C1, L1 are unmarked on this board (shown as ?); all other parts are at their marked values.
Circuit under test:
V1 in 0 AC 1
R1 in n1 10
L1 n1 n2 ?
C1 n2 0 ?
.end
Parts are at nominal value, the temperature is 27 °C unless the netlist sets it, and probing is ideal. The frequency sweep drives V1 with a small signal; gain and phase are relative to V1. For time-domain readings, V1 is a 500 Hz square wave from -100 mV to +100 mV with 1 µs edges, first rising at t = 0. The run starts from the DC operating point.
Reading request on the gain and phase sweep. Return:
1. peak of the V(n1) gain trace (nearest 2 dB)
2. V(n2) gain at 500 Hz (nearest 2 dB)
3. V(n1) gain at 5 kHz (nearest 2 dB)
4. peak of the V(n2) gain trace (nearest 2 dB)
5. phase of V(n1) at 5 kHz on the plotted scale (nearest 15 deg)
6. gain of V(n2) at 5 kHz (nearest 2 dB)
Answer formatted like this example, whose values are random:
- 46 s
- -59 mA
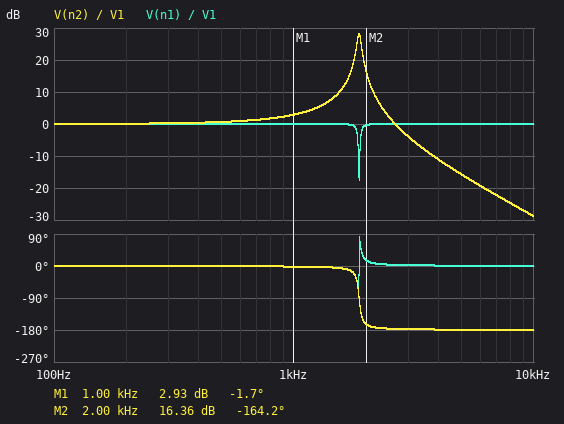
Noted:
- 0 dB
- 0 dB
- 0 dB
- 28 dB
- 0 deg
- -16 dB
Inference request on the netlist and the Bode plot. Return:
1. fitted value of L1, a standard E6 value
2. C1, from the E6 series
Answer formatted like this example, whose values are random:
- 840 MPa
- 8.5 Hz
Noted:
- 22 mH
- 330 nF
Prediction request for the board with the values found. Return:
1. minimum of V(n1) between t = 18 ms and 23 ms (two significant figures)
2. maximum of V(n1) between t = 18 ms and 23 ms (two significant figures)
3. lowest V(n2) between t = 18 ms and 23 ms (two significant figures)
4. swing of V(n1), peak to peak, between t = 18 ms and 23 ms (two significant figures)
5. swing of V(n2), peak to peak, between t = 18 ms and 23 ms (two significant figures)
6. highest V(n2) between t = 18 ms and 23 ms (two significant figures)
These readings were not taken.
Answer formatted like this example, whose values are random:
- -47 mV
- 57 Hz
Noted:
- -100 mV
- 100 mV
- -220 mV
- 210 mV
- 430 mV
- 220 mV
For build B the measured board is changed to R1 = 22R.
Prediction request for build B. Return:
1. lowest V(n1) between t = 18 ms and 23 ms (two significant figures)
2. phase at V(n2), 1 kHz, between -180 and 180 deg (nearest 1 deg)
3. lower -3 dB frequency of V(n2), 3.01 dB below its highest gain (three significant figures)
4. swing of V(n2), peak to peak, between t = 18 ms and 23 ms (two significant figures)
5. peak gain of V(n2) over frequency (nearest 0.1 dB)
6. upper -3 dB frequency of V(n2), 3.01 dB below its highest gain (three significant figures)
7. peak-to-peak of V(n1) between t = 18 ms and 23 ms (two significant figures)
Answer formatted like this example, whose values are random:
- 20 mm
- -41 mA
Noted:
- -110 mV
- -4 deg
- 1.78 kHz
- 440 mV
- 21.4 dB
- 1.94 kHz
- 220 mV
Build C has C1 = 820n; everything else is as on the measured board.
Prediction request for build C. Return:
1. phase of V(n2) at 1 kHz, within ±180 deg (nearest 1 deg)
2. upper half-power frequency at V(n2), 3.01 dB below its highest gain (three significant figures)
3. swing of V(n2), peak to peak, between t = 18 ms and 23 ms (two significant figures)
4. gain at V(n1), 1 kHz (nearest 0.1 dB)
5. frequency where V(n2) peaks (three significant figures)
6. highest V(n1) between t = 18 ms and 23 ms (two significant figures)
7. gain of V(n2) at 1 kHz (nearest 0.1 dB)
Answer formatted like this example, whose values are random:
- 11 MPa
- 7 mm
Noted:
- -10 deg
- 1.22 kHz
- 440 mV
- -0.1 dB
- 1.18 kHz
- 110 mV
- 10.7 dB
